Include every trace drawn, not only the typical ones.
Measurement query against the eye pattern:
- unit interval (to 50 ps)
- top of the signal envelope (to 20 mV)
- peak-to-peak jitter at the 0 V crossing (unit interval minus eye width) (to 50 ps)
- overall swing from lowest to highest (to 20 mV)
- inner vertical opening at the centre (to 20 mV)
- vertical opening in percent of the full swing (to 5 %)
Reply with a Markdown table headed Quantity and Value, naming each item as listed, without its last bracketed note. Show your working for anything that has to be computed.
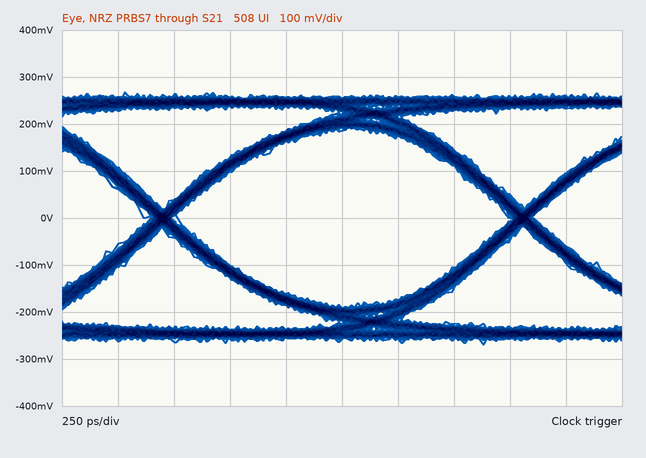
| Quantity | Value |
|---|---|
| unit interval | 1.60 ns |
| top of the signal envelope | 260 mV |
| peak-to-peak jitter at the 0 V crossing (unit interval minus eye width) | 150 ps |
| overall swing from lowest to highest | 540 mV |
| inner vertical opening at the centre | 380 mV |
| vertical opening in percent of the full swing | 380 mV / 540 mV ≈ 70 % |
